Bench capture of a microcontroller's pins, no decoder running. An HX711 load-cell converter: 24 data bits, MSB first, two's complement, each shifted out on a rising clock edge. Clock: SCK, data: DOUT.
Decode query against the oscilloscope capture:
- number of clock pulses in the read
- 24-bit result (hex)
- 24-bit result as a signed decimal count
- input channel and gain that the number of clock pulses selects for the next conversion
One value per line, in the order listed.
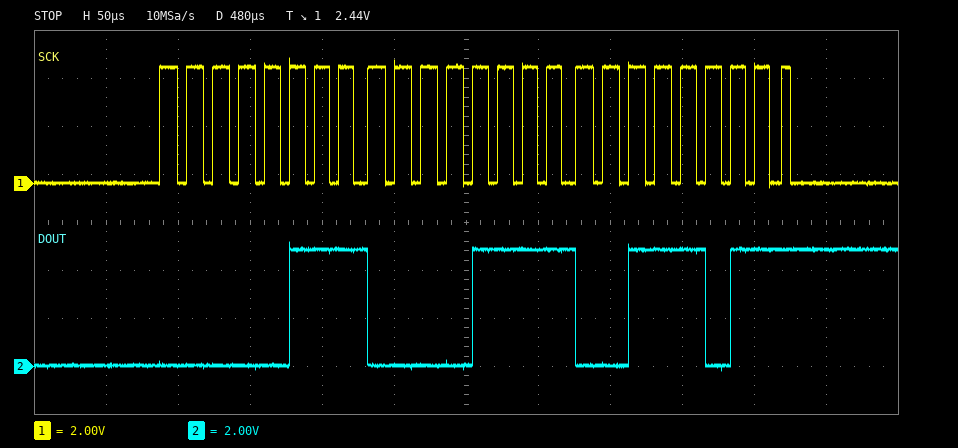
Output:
25
0x070F3B
462651
channel A, gain 128
